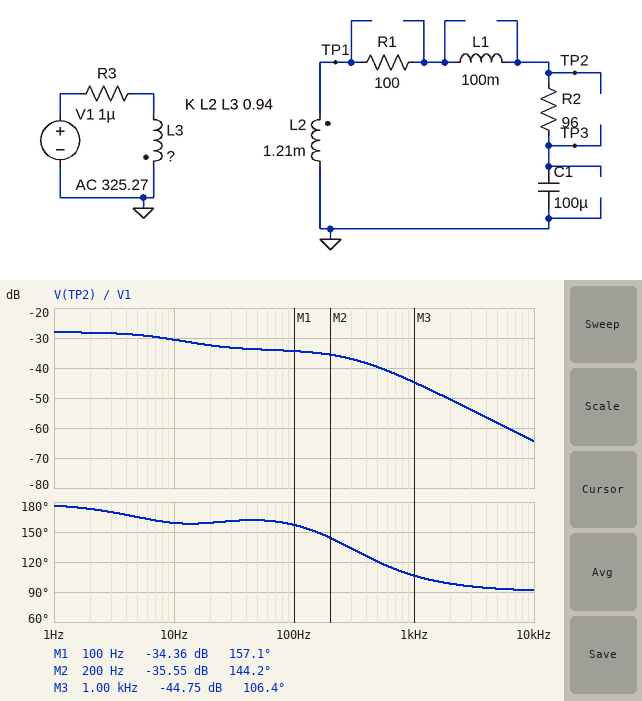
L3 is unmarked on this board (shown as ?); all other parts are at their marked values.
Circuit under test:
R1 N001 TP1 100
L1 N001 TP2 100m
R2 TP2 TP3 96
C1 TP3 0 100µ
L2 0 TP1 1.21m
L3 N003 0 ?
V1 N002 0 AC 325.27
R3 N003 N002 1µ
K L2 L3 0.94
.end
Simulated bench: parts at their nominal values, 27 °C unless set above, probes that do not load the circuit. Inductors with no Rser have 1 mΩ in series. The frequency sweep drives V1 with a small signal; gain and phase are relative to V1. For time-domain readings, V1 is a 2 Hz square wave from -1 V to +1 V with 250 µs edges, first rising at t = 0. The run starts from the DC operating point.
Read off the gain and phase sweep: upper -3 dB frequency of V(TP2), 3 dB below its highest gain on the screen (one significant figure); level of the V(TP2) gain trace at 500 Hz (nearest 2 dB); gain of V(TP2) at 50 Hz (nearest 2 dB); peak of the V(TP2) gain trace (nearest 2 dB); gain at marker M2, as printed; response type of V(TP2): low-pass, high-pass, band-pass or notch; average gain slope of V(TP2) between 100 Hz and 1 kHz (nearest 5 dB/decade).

10 Hz
-40 dB
-34 dB
-28 dB
-35.55 dB
low-pass
-10 dB/decade
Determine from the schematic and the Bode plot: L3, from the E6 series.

680 mH
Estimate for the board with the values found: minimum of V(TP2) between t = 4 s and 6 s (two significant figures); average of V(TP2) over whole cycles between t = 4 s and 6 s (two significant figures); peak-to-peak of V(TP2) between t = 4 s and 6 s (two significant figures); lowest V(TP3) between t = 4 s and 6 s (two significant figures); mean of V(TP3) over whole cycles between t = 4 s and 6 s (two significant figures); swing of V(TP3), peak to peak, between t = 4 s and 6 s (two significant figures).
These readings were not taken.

-79 mV
-39 mV
79 mV
-79 mV
-39 mV
79 mV
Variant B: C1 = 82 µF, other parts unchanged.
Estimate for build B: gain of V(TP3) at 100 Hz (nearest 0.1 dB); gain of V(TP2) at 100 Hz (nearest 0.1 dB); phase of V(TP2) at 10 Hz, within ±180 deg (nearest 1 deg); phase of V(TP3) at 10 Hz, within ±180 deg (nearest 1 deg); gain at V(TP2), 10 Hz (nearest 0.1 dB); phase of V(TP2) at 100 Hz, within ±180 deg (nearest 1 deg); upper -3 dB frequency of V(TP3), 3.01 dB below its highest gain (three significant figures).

-48.3 dB
-34.3 dB
160 deg
134 deg
-30.0 dB
156 deg
10.2 Hz
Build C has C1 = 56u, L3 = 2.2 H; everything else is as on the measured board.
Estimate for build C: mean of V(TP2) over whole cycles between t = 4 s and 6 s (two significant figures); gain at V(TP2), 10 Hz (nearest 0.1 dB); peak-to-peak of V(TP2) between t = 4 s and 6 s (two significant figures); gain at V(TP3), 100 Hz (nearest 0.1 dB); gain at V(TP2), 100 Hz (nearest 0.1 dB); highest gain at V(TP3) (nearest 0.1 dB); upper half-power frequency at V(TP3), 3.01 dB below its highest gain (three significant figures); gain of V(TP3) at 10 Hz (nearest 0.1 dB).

-22 mV
-34.2 dB
44 mV
-50.0 dB
-39.1 dB
-33.1 dB
15.2 Hz
-34.7 dB
